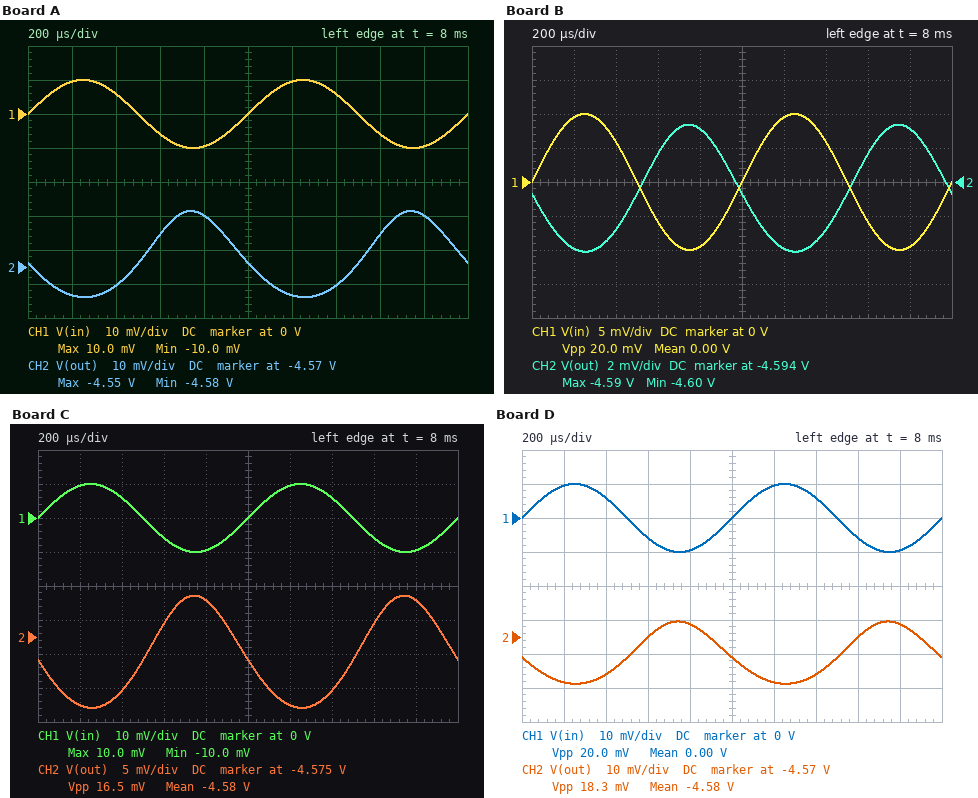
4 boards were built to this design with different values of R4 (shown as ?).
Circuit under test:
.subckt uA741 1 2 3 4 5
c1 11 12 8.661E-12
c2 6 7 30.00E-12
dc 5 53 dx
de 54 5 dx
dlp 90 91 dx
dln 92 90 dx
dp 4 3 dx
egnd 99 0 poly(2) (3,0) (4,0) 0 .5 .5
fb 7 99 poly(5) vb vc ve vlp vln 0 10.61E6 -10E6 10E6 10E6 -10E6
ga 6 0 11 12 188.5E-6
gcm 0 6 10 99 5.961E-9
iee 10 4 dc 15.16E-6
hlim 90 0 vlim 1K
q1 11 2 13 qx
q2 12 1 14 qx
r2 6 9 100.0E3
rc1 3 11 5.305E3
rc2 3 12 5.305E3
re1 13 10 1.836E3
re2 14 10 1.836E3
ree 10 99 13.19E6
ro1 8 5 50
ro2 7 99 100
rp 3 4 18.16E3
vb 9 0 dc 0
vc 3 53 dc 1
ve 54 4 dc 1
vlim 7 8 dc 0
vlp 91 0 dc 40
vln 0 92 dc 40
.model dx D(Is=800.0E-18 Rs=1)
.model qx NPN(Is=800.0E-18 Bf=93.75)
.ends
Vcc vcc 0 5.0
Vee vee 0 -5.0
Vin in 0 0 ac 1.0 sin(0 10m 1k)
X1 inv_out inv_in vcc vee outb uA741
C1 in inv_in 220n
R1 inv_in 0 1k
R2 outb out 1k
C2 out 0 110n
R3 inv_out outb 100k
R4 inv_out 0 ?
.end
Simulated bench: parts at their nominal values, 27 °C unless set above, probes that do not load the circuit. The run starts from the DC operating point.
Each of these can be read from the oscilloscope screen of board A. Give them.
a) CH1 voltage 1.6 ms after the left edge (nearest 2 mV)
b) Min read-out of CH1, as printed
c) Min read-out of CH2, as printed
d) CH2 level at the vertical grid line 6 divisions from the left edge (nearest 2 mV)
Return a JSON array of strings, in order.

["-6 mV", "-10.0 mV", "-4.58 V", "-4.578 V"]
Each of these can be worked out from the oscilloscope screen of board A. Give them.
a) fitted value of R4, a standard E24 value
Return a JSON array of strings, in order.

["330 Ω"]
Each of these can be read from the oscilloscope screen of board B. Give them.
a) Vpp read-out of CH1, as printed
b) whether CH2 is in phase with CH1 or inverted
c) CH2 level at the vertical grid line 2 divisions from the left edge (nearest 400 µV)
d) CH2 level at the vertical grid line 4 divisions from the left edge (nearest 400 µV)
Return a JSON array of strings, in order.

["20.0 mV", "inverted", "-4.5968 V", "-4.5908 V"]
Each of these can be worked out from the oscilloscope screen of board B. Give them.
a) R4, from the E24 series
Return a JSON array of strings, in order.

["910 Ω"]
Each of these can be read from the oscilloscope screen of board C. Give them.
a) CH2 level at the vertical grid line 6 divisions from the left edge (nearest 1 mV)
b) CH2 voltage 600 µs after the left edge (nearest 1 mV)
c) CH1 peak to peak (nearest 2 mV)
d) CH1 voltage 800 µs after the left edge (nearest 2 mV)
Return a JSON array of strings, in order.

["-4.585 V", "-4.573 V", "20 mV", "-10 mV"]
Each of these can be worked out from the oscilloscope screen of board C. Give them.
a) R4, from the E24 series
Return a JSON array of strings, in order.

["470 Ω"]
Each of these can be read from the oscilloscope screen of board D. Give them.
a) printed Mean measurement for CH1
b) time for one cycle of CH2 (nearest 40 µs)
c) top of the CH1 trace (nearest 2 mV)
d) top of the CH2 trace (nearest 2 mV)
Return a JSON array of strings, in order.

["0.00 V", "1.00 ms", "10 mV", "-4.566 V"]
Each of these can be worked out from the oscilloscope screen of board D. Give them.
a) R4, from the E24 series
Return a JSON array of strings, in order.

["430 Ω"]
